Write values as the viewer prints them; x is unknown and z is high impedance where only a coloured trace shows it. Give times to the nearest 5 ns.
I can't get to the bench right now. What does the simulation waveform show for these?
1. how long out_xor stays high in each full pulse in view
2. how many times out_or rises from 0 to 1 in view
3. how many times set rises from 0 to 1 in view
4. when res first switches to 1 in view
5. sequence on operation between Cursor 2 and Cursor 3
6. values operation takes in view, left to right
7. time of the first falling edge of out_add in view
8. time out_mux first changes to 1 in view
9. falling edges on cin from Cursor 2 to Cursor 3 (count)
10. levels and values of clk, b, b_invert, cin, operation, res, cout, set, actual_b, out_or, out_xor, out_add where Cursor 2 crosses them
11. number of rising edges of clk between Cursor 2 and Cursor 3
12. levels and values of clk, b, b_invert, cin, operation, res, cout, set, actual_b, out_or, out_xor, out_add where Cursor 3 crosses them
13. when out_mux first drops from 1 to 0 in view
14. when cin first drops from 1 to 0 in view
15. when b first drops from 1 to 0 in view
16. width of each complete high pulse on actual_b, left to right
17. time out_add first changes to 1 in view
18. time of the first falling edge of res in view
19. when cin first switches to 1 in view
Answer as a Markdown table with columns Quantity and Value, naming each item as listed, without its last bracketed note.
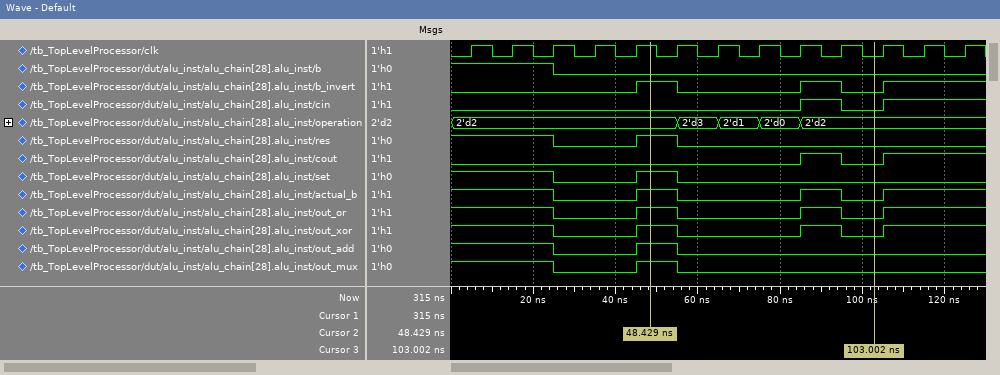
| Quantity | Value |
|---|---|
| how long out_xor stays high in each full pulse in view | 10 ns, 10 ns |
| how many times out_or rises from 0 to 1 in view | 3 |
| how many times set rises from 0 to 1 in view | 1 |
| when res first switches to 1 in view | 45 ns |
| sequence on operation between Cursor 2 and Cursor 3 | 2'd2, 2'd3, 2'd1, 2'd0, 2'd2 |
| values operation takes in view, left to right | 2'd2, 2'd3, 2'd1, 2'd0, 2'd2 |
| time of the first falling edge of out_add in view | 25 ns |
| time out_mux first changes to 1 in view | 45 ns |
| falling edges on cin from Cursor 2 to Cursor 3 | 1 |
| levels and values of clk, b, b_invert, cin, operation, res, cout, set, actual_b, out_or, out_xor, out_add where Cursor 2 crosses them | clk=1, b=0, b_invert=1, cin=0, operation=2'd2, res=1, cout=0, set=1, actual_b=1, out_or=1, out_xor=1, out_add=1 |
| number of rising edges of clk between Cursor 2 and Cursor 3 | 5 |
| levels and values of clk, b, b_invert, cin, operation, res, cout, set, actual_b, out_or, out_xor, out_add where Cursor 3 crosses them | clk=0, b=0, b_invert=0, cin=0, operation=2'd2, res=0, cout=0, set=0, actual_b=0, out_or=0, out_xor=0, out_add=0 |
| when out_mux first drops from 1 to 0 in view | 25 ns |
| when cin first drops from 1 to 0 in view | 95 ns |
| when b first drops from 1 to 0 in view | 25 ns |
| width of each complete high pulse on actual_b, left to right | 10 ns, 10 ns |
| time out_add first changes to 1 in view | 45 ns |
| time of the first falling edge of res in view | 25 ns |
| when cin first switches to 1 in view | 85 ns |
